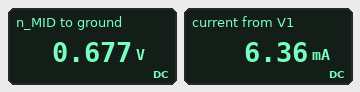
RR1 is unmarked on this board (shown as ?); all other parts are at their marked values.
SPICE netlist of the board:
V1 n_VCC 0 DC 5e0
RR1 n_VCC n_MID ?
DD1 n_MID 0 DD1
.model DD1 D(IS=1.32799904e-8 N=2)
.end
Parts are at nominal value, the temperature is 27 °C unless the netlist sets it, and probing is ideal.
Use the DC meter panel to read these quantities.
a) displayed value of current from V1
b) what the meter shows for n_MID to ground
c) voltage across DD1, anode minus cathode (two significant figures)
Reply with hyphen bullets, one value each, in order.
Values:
- 6.36 mA
- 0.677 V
- 680 mV
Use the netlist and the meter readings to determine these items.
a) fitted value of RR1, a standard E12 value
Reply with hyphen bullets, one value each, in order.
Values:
- 680 Ω
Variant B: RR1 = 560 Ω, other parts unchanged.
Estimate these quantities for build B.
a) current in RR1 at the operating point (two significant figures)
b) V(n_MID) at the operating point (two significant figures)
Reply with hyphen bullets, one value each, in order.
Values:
- 7.7 mA
- 690 mV
